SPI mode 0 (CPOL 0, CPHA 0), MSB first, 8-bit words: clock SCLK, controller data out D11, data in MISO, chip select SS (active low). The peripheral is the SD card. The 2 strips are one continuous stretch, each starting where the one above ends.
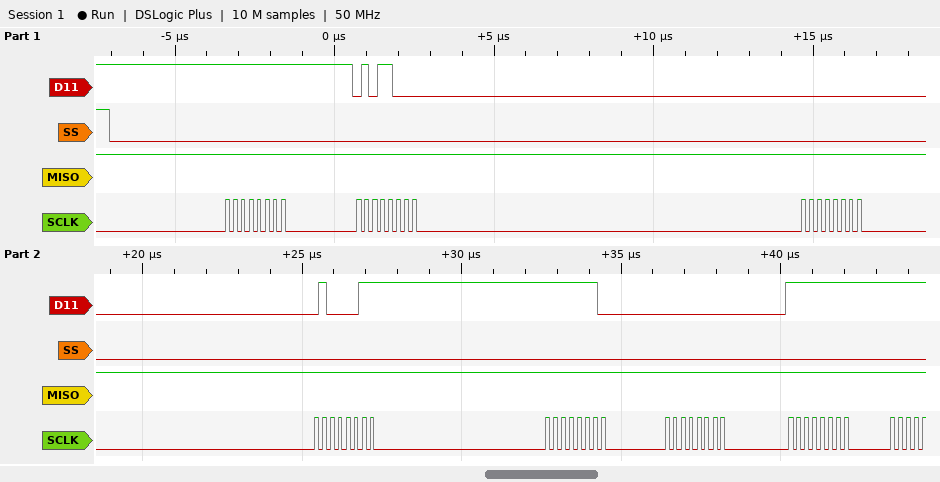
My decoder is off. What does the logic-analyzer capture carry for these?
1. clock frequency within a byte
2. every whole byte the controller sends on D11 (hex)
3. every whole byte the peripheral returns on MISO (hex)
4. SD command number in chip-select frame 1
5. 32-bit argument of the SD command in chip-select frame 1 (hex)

4 MHz
FF 58 00 43 FE 00 FF
FF FF FF FF FF FF FF
CMD24
0x0043FE00
